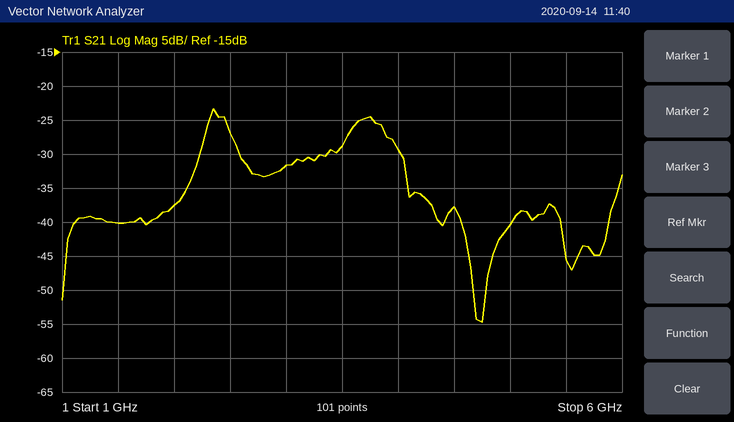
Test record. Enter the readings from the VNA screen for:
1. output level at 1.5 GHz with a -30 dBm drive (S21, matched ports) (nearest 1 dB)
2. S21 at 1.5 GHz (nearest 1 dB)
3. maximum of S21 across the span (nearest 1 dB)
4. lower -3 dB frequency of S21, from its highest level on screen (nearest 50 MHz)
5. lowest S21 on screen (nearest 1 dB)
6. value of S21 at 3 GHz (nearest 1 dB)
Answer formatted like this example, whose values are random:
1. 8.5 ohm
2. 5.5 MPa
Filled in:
1. -70 dBm
2. -40 dB
3. -23 dB
4. 2.30 GHz
5. -55 dB
6. -32 dB
